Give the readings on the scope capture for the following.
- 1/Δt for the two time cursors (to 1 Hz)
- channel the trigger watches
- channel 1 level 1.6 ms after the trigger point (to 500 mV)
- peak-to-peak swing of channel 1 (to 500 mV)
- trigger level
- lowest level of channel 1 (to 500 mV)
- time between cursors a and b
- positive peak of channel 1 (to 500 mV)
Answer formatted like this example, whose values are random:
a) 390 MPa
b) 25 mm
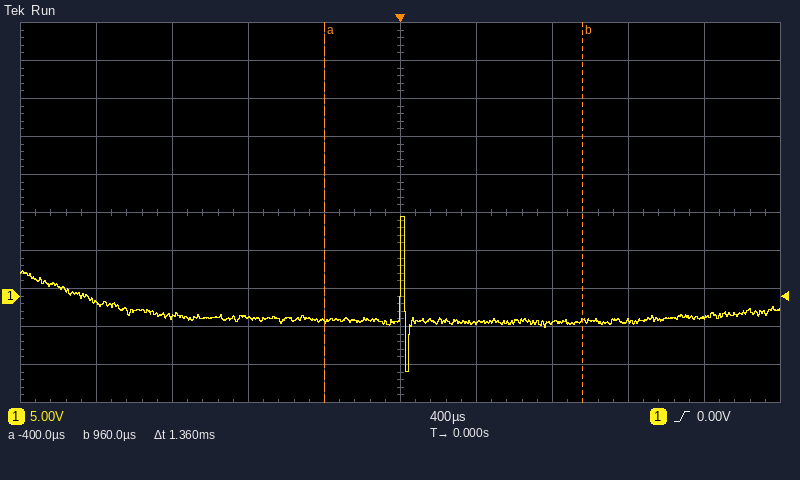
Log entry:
a) 735 Hz
b) channel 1
c) -3.0 V
d) 20.5 V
e) 0.00 V
f) -10.0 V
g) 1.36 ms
h) 10.5 V
